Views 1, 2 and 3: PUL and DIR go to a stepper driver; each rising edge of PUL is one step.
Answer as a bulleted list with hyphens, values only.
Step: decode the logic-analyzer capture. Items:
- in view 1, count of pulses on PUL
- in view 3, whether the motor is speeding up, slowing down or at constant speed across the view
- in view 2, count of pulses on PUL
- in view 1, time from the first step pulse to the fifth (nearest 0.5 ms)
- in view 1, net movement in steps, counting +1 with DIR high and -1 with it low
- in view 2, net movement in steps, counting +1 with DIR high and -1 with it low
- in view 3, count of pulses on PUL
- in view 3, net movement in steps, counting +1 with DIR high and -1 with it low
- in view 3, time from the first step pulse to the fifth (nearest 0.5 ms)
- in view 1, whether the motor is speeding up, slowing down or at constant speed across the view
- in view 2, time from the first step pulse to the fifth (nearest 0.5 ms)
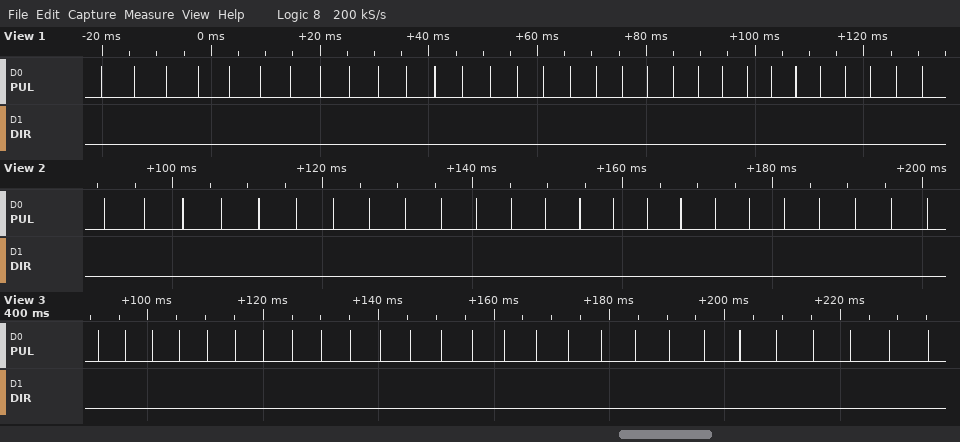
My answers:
- 31
- slowing down
- 24
- 23.5 ms
- -31
- -24
- 27
- -27
- 19.0 ms
- speeding up
- 20.5 ms
